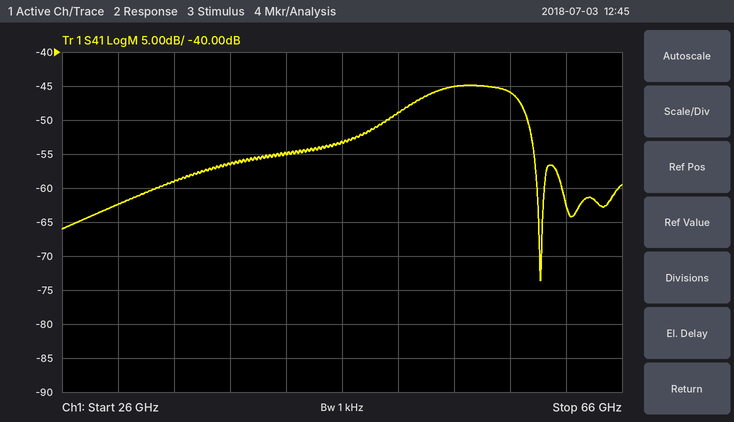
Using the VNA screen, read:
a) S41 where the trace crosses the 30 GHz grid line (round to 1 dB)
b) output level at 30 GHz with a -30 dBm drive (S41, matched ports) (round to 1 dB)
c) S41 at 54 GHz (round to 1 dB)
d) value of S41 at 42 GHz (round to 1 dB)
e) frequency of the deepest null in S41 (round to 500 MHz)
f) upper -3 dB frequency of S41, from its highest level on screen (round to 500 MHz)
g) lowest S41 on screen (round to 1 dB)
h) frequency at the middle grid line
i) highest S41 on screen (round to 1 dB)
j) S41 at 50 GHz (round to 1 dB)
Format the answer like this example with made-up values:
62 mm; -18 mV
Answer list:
-62 dB; -92 dBm; -45 dB; -55 dB; 60.0 GHz; 59.0 GHz; -74 dB; 46 GHz; -45 dB; -49 dB
